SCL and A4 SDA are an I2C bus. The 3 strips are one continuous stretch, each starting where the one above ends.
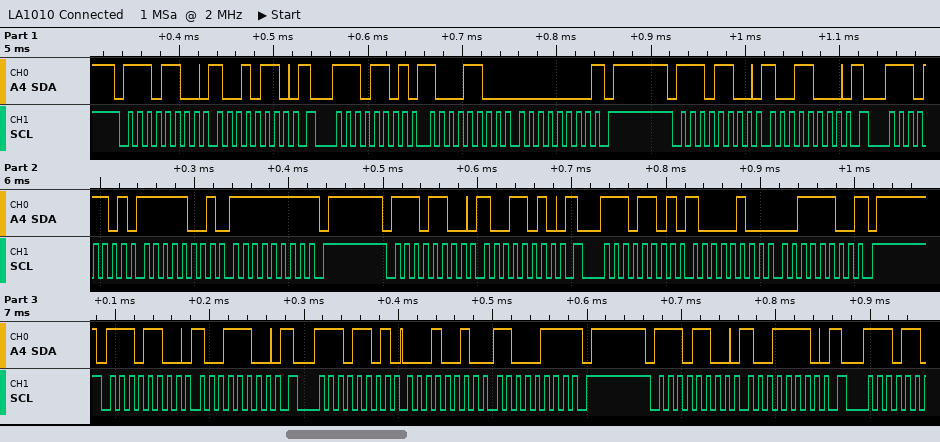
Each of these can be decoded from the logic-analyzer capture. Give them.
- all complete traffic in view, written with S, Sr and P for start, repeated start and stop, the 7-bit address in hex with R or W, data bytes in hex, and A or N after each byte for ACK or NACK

S 76W A 96 A Sr 76R A 8C A 00 N P S 76W A 98 A Sr 76R A F9 A FF N P S 76W A 9A A Sr 76R A 84 A 3C N P S 76W A 9C A Sr 76R A 12 A C7 N P S 76W A 9E A
